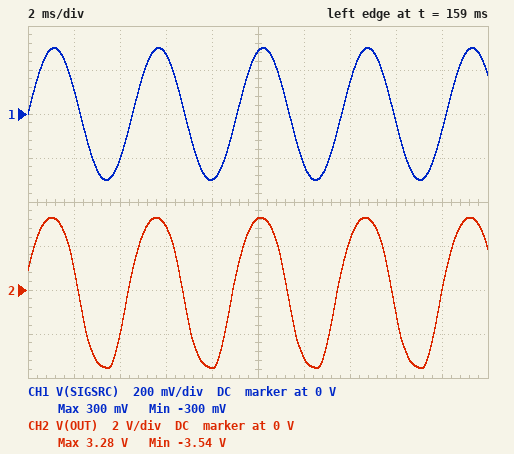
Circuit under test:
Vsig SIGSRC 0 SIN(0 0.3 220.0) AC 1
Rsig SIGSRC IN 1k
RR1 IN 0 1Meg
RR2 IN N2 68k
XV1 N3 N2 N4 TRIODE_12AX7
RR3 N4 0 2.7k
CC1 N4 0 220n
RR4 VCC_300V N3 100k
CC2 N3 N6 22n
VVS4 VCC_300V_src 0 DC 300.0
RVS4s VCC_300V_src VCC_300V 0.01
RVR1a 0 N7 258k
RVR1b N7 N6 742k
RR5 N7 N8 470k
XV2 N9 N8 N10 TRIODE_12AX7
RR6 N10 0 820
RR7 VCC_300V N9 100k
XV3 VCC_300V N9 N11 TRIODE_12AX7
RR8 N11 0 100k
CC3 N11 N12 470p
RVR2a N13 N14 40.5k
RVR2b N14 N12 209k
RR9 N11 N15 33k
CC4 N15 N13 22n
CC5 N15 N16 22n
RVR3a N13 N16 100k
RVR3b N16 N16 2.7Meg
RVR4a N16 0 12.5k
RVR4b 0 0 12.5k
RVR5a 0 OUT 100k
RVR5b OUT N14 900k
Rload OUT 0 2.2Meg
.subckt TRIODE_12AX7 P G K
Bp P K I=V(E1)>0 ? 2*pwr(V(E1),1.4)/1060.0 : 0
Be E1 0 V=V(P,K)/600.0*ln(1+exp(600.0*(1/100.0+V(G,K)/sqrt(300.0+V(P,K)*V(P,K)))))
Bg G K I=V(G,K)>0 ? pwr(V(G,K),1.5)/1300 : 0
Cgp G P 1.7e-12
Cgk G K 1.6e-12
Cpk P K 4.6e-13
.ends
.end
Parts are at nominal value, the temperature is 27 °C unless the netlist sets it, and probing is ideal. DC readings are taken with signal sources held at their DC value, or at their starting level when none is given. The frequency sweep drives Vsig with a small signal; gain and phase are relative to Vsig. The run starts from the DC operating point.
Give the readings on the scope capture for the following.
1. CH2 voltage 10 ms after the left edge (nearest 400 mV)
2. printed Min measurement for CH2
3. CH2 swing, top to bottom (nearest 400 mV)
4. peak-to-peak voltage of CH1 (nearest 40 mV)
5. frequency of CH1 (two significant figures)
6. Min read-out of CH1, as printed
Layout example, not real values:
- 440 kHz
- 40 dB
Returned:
- 3.2 V
- -3.54 V
- 6.8 V
- 600 mV
- 220 Hz
- -300 mV
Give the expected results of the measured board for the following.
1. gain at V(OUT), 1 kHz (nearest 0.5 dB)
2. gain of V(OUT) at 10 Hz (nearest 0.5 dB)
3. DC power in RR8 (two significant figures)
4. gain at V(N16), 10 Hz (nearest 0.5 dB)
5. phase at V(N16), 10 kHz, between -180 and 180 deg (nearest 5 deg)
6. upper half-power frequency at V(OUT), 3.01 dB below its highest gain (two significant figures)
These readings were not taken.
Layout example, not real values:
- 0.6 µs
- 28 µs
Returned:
- 24.0 dB
- 8.5 dB
- 310 mW
- 15.5 dB
- -90 deg
- 4.8 kHz
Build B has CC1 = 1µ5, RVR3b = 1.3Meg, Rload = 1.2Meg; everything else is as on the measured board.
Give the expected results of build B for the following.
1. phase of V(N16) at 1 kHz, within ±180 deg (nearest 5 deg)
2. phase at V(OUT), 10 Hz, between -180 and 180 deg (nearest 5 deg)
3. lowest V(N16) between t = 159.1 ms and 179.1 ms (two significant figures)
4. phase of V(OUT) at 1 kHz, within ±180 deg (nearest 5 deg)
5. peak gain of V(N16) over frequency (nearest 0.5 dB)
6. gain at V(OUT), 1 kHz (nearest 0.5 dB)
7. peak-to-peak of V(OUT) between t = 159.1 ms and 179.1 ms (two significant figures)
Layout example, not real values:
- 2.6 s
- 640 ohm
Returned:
- -5 deg
- 120 deg
- -17 V
- -20 deg
- 43.5 dB
- 25.0 dB
- 7.6 V
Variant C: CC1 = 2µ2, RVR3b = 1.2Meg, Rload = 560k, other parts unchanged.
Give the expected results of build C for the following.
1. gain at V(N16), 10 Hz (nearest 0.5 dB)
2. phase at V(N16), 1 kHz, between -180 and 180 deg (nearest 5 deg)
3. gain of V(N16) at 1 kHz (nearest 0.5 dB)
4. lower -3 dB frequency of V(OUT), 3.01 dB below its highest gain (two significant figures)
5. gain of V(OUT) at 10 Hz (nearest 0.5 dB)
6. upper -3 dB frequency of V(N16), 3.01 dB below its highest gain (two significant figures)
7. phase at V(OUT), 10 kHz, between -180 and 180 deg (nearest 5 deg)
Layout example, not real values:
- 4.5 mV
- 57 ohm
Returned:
- 16.0 dB
- -5 deg
- 43.5 dB
- 60 Hz
- 8.0 dB
- 3.9 kHz
- -95 deg
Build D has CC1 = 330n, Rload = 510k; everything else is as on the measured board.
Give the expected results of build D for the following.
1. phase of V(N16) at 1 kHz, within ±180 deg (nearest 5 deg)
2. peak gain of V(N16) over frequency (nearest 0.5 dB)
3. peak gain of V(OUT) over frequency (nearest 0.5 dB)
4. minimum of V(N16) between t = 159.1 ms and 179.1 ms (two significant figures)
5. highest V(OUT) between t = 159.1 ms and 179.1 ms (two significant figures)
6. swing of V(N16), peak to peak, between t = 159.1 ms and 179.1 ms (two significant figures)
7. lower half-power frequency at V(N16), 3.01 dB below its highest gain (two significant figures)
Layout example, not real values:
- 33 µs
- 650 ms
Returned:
- 5 deg
- 43.0 dB
- 24.0 dB
- -15 V
- 3.1 V
- 29 V
- 410 Hz
